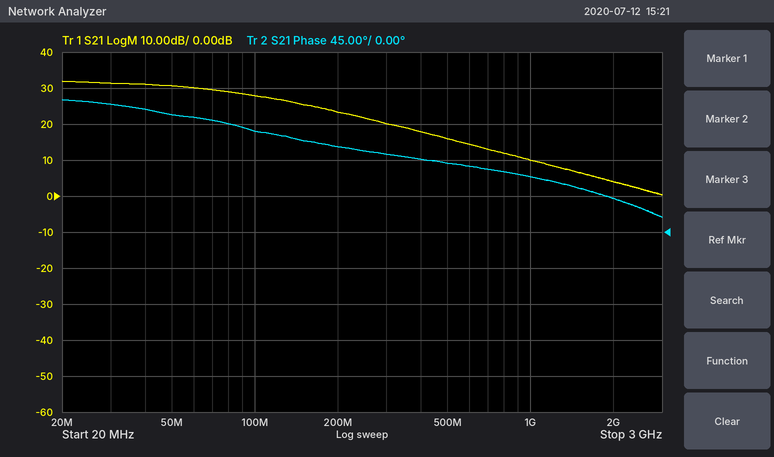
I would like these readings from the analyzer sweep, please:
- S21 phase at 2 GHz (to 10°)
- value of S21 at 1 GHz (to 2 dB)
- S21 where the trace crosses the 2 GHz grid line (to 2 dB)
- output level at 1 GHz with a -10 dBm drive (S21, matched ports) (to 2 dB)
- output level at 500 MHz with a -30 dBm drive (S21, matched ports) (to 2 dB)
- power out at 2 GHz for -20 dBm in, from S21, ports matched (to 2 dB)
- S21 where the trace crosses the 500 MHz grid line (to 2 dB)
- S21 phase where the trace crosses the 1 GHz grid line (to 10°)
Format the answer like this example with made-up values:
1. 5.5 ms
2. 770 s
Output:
1. 40°
2. 10 dB
3. 4 dB
4. 0 dBm
5. -14 dBm
6. -16 dBm
7. 16 dB
8. 70°
